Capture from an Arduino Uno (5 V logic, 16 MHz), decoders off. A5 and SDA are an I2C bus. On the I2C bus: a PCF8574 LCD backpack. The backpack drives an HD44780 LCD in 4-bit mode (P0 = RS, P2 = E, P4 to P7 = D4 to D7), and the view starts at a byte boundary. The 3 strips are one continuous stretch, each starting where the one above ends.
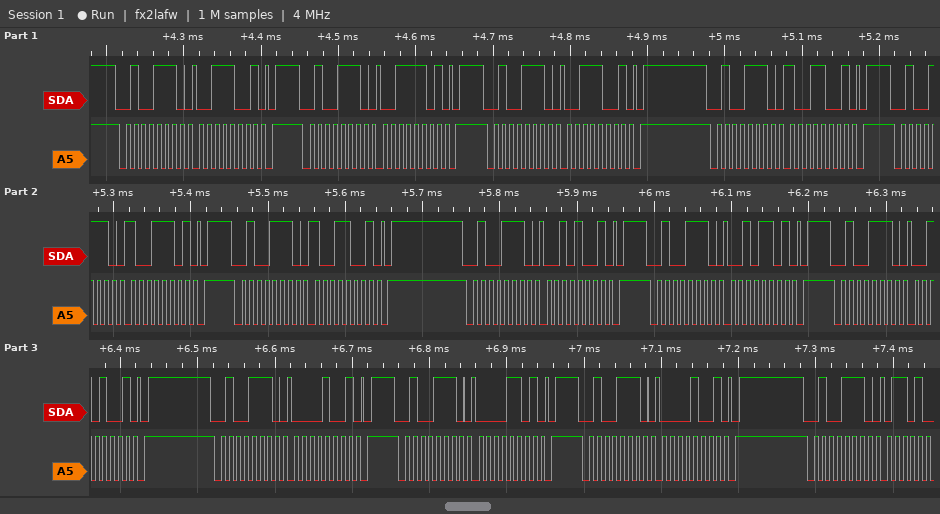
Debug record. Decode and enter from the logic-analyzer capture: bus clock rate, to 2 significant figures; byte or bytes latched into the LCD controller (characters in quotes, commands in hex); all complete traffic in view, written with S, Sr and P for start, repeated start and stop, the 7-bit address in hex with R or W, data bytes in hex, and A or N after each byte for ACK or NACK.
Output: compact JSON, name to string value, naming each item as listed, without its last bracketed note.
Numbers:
{"bus clock rate, to 2 significant figures": "100 kHz", "byte or bytes latched into the LCD controller": "'9' ' '", "all complete traffic in view, written with S, Sr and P for start, repeated start and stop, the 7-bit address in hex with R or W, data bytes in hex, and A or N after each byte for ACK or NACK": "S 27W A 39 A P S 27W A 3D A P S 27W A 39 A P S 27W A 99 A P S 27W A 9D A P S 27W A 99 A P S 27W A 29 A P S 27W A 2D A P S 27W A 29 A P S 27W A 09 A P S 27W A 0D A P S 27W A 09 A P S 27W A"}
